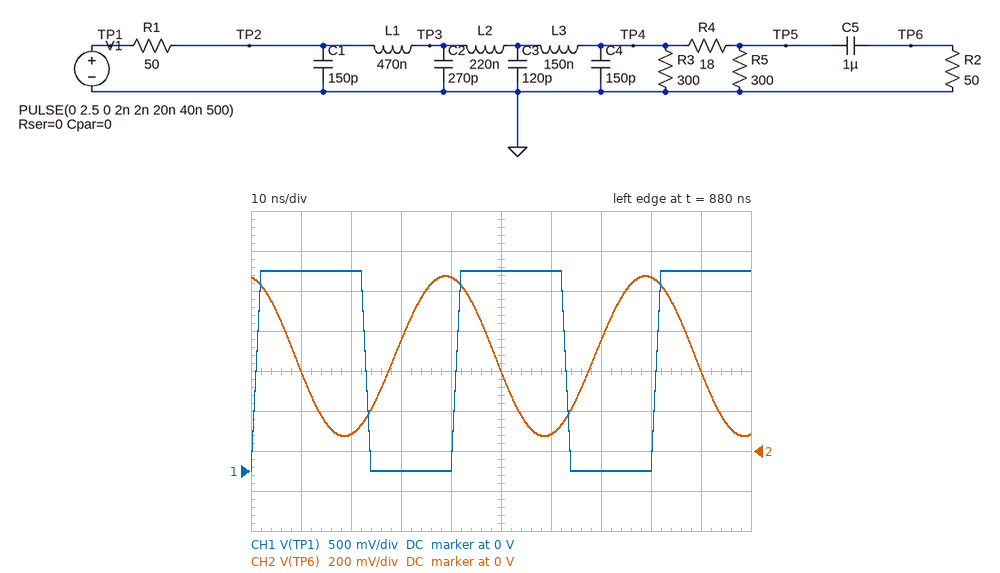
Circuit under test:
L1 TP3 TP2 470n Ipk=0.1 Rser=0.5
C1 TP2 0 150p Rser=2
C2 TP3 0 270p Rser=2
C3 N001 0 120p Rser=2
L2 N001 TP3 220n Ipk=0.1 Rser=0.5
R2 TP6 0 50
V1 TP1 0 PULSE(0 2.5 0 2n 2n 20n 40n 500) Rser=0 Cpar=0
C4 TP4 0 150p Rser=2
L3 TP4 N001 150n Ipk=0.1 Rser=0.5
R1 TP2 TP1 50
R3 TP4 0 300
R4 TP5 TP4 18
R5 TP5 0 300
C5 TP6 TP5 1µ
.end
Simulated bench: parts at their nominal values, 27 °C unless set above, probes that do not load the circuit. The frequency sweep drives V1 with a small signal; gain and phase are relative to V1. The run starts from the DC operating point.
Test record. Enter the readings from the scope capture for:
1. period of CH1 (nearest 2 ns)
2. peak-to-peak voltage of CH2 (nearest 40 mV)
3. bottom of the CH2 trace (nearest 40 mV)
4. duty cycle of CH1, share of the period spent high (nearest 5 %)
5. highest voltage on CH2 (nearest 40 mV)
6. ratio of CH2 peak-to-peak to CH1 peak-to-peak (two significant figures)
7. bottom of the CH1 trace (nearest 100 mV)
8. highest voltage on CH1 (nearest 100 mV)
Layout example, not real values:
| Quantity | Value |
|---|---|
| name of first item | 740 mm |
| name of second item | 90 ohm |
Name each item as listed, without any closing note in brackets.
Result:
| Quantity | Value |
|---|---|
| period of CH1 | 40 ns |
| peak-to-peak voltage of CH2 | 800 mV |
| bottom of the CH2 trace | 80 mV |
| duty cycle of CH1, share of the period spent high | 55 % |
| highest voltage on CH2 | 880 mV |
| ratio of CH2 peak-to-peak to CH1 peak-to-peak | 0.32 |
| bottom of the CH1 trace | 0 V |
| highest voltage on CH1 | 2.5 V |
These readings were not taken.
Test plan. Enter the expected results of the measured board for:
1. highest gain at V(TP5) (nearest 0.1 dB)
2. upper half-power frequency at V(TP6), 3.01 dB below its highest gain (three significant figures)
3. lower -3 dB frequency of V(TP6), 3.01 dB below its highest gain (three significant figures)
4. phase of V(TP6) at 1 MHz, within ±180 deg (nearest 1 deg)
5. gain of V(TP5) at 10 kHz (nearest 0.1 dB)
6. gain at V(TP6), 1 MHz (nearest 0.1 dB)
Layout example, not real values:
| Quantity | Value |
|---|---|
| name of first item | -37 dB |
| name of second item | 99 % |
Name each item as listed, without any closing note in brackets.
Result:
| Quantity | Value |
|---|---|
| highest gain at V(TP5) | -3.0 dB |
| upper half-power frequency at V(TP6), 3.01 dB below its highest gain | 25.8 MHz |
| lower -3 dB frequency of V(TP6), 3.01 dB below its highest gain | 1.57 kHz |
| phase of V(TP6) at 1 MHz, within ±180 deg | -9 deg |
| gain of V(TP5) at 10 kHz | -8.8 dB |
| gain at V(TP6), 1 MHz | -9.2 dB |
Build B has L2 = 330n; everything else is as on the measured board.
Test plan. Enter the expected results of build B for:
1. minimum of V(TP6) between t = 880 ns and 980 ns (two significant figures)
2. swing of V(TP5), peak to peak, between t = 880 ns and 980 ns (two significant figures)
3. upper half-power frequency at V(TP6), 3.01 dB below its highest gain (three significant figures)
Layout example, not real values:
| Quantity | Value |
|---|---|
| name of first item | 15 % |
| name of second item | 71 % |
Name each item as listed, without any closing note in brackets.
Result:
| Quantity | Value |
|---|---|
| minimum of V(TP6) between t = 880 ns and 980 ns | 90 mV |
| swing of V(TP5), peak to peak, between t = 880 ns and 980 ns | 770 mV |
| upper half-power frequency at V(TP6), 3.01 dB below its highest gain | 25.0 MHz |
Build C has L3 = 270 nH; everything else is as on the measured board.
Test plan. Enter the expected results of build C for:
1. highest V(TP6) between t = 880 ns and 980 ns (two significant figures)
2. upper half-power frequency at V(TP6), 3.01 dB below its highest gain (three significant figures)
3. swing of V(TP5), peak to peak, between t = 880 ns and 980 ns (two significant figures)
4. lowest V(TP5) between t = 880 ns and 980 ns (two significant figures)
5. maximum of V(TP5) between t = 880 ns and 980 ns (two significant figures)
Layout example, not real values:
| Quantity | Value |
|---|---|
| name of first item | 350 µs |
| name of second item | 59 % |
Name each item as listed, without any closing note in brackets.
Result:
| Quantity | Value |
|---|---|
| highest V(TP6) between t = 880 ns and 980 ns | 840 mV |
| upper half-power frequency at V(TP6), 3.01 dB below its highest gain | 24.5 MHz |
| swing of V(TP5), peak to peak, between t = 880 ns and 980 ns | 730 mV |
| lowest V(TP5) between t = 880 ns and 980 ns | 110 mV |
| maximum of V(TP5) between t = 880 ns and 980 ns | 850 mV |
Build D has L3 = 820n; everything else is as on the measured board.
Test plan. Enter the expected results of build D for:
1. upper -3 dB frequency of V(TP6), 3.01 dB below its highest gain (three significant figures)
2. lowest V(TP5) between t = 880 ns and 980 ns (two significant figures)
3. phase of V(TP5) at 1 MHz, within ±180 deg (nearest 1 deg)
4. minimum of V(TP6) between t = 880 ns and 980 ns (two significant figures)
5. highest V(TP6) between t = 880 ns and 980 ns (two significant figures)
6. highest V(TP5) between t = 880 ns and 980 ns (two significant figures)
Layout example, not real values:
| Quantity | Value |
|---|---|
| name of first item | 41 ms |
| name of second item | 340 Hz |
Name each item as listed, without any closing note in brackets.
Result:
| Quantity | Value |
|---|---|
| upper -3 dB frequency of V(TP6), 3.01 dB below its highest gain | 17.0 MHz |
| lowest V(TP5) between t = 880 ns and 980 ns | 350 mV |
| phase of V(TP5) at 1 MHz, within ±180 deg | -12 deg |
| minimum of V(TP6) between t = 880 ns and 980 ns | 340 mV |
| highest V(TP6) between t = 880 ns and 980 ns | 610 mV |
| highest V(TP5) between t = 880 ns and 980 ns | 620 mV |
